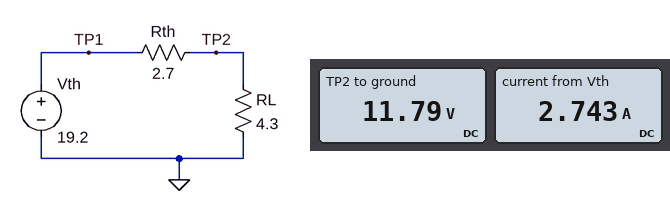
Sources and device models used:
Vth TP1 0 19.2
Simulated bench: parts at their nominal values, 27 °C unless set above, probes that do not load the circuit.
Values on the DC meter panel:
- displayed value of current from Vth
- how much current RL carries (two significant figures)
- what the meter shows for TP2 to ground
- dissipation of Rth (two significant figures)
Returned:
2.743 A
2.7 A
11.79 V
20 W
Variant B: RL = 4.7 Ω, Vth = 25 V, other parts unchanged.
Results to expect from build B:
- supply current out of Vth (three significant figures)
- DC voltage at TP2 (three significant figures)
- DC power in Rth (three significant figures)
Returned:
3.38 A
15.9 V
30.8 W
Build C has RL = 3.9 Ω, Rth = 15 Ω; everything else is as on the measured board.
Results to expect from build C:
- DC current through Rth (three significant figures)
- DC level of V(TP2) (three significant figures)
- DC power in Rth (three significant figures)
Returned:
1.02 A
3.96 V
15.5 W
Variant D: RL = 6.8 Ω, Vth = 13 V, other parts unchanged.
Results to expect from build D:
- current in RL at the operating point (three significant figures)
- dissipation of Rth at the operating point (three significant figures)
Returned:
1.37 A
5.06 W
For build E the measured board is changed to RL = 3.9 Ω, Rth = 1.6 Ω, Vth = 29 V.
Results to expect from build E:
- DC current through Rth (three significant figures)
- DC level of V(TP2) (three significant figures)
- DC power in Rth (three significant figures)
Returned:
5.27 A
20.6 V
44.5 W
